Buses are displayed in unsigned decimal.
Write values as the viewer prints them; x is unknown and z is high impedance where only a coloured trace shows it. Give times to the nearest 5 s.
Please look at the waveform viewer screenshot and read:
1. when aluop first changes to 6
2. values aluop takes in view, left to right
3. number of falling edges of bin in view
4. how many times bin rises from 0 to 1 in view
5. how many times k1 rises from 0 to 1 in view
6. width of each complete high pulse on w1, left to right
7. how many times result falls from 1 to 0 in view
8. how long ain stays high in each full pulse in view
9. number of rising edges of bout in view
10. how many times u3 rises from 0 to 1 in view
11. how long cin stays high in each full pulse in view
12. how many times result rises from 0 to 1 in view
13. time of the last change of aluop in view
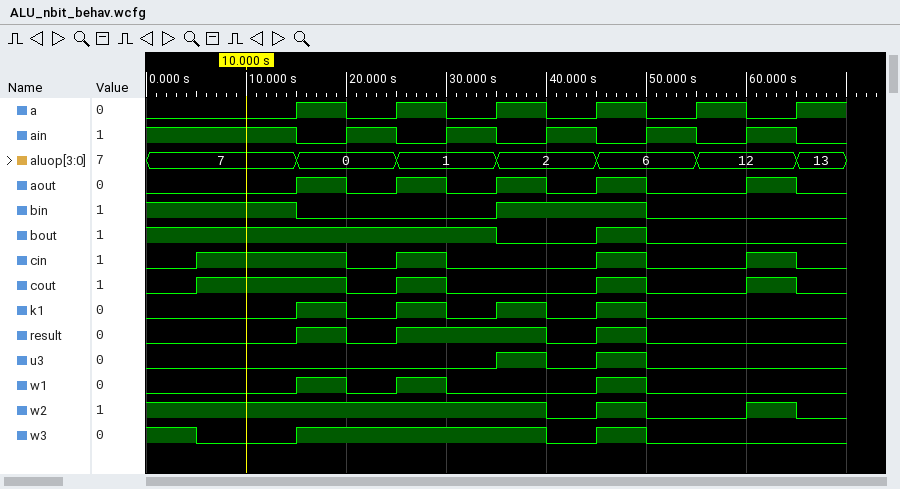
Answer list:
45 s
7, 0, 1, 2, 6, 12, 13
2
1
4
5 s, 5 s, 5 s
3
5 s, 5 s, 5 s, 5 s, 5 s
1
2
15 s, 5 s, 5 s, 5 s
3
65 s
